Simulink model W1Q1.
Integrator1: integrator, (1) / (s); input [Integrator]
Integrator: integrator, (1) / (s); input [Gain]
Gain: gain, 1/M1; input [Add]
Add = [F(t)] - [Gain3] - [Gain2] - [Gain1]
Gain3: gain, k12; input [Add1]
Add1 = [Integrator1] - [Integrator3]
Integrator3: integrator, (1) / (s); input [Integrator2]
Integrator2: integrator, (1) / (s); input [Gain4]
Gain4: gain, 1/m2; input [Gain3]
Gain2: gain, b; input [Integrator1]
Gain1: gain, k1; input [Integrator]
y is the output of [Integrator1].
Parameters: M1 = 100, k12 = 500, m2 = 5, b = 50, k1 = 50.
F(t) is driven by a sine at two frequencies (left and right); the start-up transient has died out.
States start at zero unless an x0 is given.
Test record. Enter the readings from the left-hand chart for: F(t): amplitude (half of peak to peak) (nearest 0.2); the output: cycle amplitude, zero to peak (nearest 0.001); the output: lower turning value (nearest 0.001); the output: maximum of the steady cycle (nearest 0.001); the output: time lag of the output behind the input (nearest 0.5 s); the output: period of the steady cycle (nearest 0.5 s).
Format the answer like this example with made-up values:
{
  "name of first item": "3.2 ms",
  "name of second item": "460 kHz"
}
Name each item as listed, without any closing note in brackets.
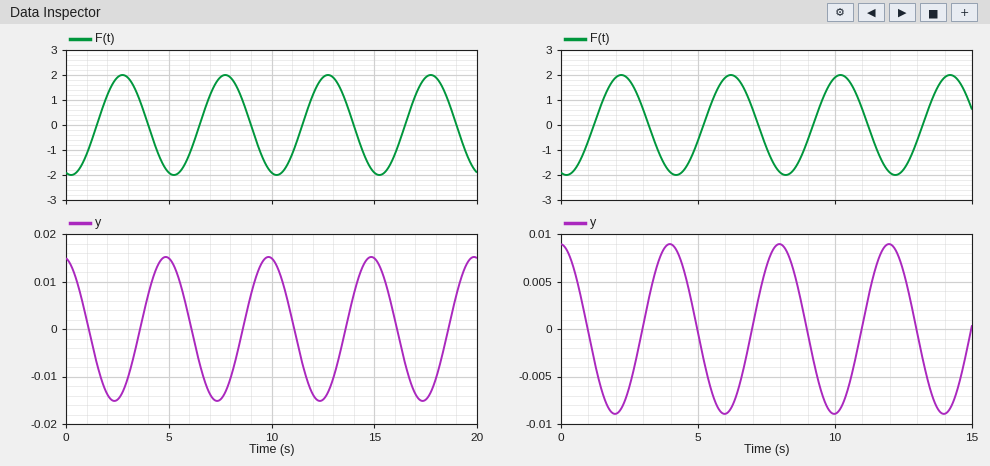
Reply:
{
  "F(t): amplitude (half of peak to peak)": "2.0",
  "the output: cycle amplitude, zero to peak": "0.015",
  "the output: lower turning value": "-0.015",
  "the output: maximum of the steady cycle": "0.015",
  "the output: time lag of the output behind the input": "2.0 s",
  "the output: period of the steady cycle": "5.0 s"
}
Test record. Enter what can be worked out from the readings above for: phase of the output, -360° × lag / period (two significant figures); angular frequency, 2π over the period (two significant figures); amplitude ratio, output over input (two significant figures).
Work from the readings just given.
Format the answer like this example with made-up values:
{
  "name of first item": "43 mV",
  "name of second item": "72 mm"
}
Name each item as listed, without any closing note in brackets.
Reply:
{
  "phase of the output, -360° × lag / period": "-140°",
  "angular frequency, 2π over the period": "1.3 rad/s",
  "amplitude ratio, output over input": "0.0075"
}
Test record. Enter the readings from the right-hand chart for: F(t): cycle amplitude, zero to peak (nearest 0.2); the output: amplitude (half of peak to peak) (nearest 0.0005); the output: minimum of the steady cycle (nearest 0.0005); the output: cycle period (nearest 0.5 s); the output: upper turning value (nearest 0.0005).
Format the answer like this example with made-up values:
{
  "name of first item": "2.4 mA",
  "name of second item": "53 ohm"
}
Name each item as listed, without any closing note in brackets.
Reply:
{
  "F(t): cycle amplitude, zero to peak": "2.0",
  "the output: amplitude (half of peak to peak)": "0.0090",
  "the output: minimum of the steady cycle": "-0.0090",
  "the output: cycle period": "4.0 s",
  "the output: upper turning value": "0.0090"
}
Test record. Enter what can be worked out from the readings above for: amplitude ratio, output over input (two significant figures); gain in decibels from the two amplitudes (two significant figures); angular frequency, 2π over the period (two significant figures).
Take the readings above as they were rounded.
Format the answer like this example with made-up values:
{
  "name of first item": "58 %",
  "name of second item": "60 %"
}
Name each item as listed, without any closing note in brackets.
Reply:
{
  "amplitude ratio, output over input": "0.0045",
  "gain in decibels from the two amplitudes": "-47 dB",
  "angular frequency, 2π over the period": "1.6 rad/s"
}
